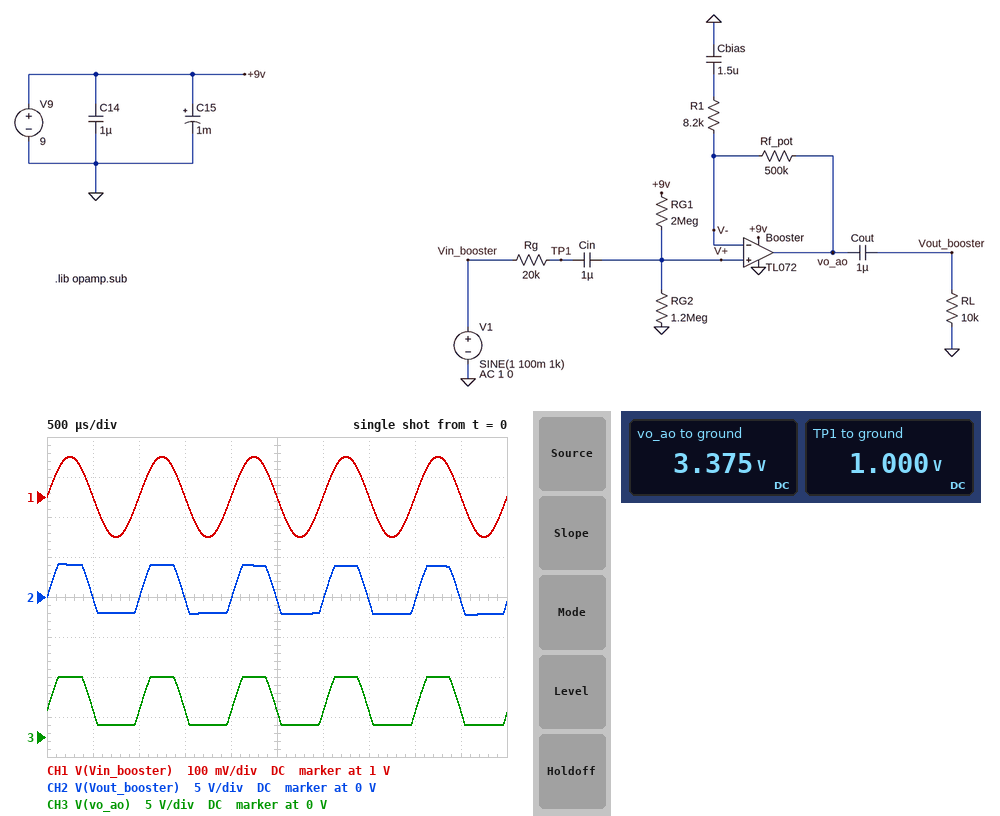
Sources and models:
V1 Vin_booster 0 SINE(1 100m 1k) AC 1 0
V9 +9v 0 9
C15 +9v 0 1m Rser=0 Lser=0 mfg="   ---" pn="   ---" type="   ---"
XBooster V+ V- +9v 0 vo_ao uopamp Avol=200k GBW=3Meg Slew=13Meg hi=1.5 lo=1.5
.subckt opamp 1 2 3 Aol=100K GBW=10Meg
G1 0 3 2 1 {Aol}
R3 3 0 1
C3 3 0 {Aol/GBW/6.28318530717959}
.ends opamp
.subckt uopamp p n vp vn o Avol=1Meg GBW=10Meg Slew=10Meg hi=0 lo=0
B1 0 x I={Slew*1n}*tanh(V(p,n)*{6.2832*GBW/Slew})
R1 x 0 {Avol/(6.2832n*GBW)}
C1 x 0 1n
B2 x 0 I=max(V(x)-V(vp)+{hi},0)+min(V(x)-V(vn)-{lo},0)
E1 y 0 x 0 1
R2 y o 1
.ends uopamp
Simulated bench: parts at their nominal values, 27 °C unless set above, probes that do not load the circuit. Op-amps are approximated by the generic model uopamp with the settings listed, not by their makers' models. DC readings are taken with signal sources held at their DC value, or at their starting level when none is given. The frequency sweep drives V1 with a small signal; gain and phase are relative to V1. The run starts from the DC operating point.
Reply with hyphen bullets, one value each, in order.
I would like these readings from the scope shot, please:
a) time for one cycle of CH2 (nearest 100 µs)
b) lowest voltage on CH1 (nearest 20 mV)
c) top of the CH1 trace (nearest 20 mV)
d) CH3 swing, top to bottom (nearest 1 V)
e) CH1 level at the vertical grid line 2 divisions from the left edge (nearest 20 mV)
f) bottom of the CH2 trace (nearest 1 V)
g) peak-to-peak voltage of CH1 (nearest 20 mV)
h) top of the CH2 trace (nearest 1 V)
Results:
- 1.0 ms
- 900 mV
- 1.10 V
- 6 V
- 1.00 V
- -2 V
- 200 mV
- 4 V
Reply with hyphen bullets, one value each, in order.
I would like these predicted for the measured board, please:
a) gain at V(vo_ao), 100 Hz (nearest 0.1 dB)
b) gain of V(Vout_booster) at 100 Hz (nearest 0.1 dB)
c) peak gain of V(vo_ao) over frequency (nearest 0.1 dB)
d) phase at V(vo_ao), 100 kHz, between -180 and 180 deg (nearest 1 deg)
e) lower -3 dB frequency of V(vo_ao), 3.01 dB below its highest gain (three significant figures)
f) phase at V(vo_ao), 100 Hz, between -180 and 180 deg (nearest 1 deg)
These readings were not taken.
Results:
- 35.5 dB
- 35.4 dB
- 35.6 dB
- -64 deg
- 12.9 Hz
- 7 deg
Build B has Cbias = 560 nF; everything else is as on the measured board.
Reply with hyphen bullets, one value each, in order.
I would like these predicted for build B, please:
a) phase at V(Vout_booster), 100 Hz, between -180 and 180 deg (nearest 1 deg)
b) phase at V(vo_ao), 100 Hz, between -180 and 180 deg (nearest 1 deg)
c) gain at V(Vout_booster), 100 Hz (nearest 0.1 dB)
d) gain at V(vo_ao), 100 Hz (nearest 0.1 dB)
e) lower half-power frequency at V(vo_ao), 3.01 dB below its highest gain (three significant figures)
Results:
- 28 deg
- 19 deg
- 35.0 dB
- 35.1 dB
- 34.6 Hz
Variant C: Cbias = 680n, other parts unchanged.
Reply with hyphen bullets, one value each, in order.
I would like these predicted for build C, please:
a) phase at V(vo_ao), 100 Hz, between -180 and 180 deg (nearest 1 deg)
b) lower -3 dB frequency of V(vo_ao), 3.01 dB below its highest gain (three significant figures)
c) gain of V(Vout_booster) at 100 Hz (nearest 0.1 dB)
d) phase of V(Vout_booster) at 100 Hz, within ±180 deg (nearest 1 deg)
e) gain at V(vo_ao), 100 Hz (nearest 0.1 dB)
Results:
- 16 deg
- 28.5 Hz
- 35.2 dB
- 25 deg
- 35.3 dB
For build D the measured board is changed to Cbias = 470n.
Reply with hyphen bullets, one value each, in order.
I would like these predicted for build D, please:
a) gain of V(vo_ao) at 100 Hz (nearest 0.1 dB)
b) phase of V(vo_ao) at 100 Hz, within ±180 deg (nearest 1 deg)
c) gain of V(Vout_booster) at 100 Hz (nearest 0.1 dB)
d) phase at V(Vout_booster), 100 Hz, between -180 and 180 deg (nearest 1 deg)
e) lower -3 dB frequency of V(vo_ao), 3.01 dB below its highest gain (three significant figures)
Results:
- 34.9 dB
- 22 deg
- 34.8 dB
- 31 deg
- 41.2 Hz
